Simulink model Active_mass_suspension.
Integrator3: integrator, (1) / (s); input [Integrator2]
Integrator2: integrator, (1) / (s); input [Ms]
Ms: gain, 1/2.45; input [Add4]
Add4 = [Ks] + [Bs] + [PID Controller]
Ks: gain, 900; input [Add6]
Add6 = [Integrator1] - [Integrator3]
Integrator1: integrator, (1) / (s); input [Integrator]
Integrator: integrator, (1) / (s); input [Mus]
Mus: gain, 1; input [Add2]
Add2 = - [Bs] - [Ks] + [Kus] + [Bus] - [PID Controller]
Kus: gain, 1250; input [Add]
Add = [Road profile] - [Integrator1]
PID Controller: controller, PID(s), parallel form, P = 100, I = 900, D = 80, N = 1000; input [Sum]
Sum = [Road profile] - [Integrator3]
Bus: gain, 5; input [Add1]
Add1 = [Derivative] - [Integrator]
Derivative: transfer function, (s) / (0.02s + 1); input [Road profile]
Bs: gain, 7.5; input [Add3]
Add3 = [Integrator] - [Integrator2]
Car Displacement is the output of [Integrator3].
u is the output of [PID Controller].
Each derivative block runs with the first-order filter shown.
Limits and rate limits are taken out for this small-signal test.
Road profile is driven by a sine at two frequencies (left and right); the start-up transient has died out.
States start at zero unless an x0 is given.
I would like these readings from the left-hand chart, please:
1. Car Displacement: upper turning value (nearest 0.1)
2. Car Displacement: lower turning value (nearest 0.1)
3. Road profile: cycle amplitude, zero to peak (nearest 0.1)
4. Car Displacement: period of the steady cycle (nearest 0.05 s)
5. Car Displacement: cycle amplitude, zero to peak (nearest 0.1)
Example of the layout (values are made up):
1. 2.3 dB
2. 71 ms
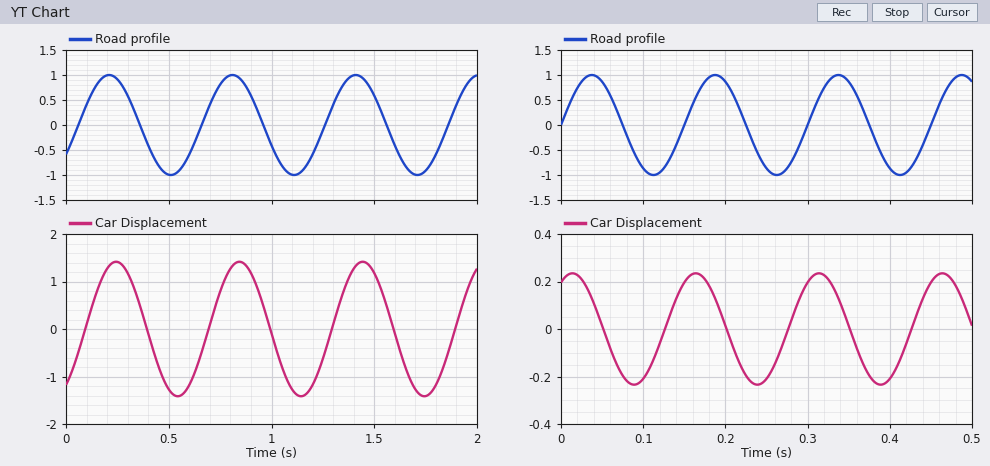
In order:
1. 1.4
2. -1.4
3. 1.0
4. 0.60 s
5. 1.4
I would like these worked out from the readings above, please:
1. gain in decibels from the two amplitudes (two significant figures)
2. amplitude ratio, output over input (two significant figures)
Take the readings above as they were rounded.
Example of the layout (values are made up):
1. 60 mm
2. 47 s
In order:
1. 2.9 dB
2. 1.4
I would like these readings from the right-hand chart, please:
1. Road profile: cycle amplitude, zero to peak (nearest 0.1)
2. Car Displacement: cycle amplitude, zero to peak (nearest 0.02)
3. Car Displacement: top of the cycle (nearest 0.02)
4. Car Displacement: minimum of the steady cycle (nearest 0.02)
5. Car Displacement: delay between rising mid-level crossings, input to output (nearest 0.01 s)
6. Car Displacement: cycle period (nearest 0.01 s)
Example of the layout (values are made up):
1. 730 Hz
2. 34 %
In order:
1. 1.0
2. 0.24
3. 0.24
4. -0.24
5. 0.13 s
6. 0.15 s
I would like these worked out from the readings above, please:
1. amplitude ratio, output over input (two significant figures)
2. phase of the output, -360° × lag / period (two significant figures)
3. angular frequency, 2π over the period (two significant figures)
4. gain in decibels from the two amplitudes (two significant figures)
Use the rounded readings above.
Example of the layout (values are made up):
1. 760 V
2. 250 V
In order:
1. 0.24
2. -310°
3. 42 rad/s
4. -12 dB
